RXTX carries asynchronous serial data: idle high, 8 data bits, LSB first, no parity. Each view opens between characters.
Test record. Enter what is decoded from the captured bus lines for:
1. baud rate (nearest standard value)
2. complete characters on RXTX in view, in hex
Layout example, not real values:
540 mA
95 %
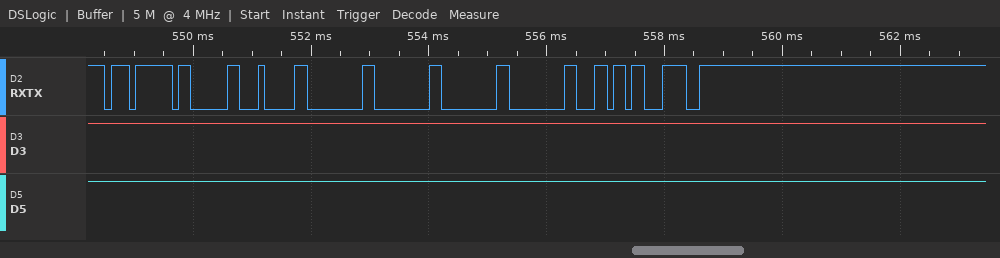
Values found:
9600 baud
F7, 03, 04, 00, 00, 00, 00, 6C, 3C
